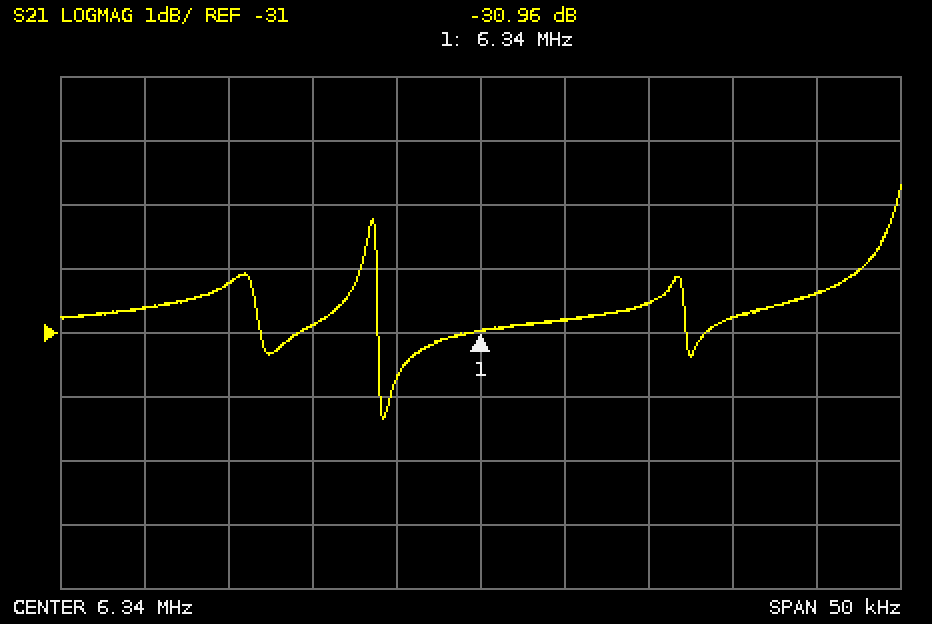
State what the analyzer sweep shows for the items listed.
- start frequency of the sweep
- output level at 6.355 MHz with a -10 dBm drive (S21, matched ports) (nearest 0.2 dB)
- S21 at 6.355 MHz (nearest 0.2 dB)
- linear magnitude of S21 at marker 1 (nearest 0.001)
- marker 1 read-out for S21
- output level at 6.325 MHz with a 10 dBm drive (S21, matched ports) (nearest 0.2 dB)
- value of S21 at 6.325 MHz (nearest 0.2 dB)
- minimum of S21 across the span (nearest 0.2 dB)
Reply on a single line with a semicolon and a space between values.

6.315 MHz; -40.8 dBm; -30.8 dB; 0.028; -30.96 dB; -20.2 dBm; -30.2 dB; -32.4 dB
